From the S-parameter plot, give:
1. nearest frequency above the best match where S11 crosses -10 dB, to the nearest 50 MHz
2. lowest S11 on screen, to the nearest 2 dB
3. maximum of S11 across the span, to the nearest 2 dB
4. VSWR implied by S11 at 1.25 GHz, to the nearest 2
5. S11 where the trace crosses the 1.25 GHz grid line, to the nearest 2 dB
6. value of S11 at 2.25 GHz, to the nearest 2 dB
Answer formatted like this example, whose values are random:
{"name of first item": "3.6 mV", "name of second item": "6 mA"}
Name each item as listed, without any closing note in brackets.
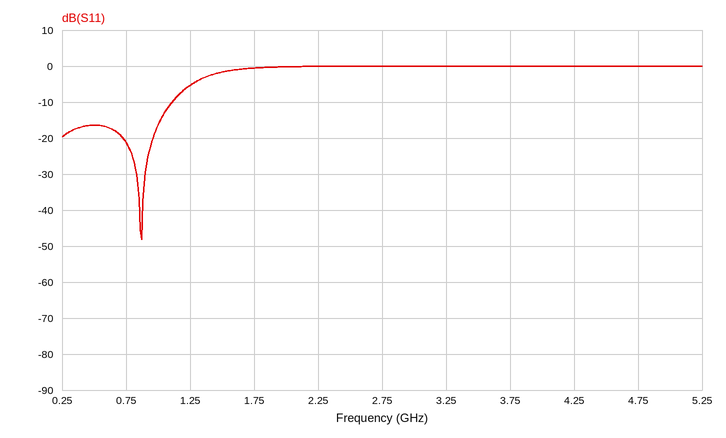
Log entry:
{"nearest frequency above the best match where S11 crosses -10 dB, to the nearest 50 MHz": "1.10 GHz", "lowest S11 on screen, to the nearest 2 dB": "-48 dB", "maximum of S11 across the span, to the nearest 2 dB": "0 dB", "VSWR implied by S11 at 1.25 GHz, to the nearest 2": "4", "S11 where the trace crosses the 1.25 GHz grid line, to the nearest 2 dB": "-6 dB", "value of S11 at 2.25 GHz, to the nearest 2 dB": "0 dB"}
